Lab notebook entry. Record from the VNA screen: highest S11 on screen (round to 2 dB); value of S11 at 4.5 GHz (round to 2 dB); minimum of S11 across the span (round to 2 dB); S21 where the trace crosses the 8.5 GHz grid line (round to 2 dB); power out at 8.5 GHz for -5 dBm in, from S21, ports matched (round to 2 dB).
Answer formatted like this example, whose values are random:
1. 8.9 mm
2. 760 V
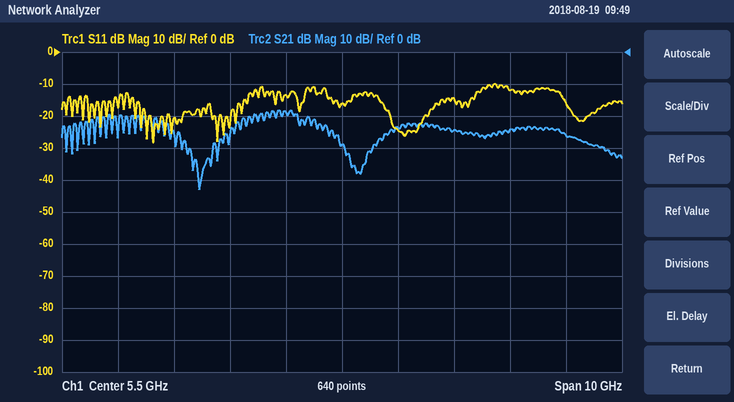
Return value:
1. -10 dB
2. -14 dB
3. -28 dB
4. -24 dB
5. -30 dBm
